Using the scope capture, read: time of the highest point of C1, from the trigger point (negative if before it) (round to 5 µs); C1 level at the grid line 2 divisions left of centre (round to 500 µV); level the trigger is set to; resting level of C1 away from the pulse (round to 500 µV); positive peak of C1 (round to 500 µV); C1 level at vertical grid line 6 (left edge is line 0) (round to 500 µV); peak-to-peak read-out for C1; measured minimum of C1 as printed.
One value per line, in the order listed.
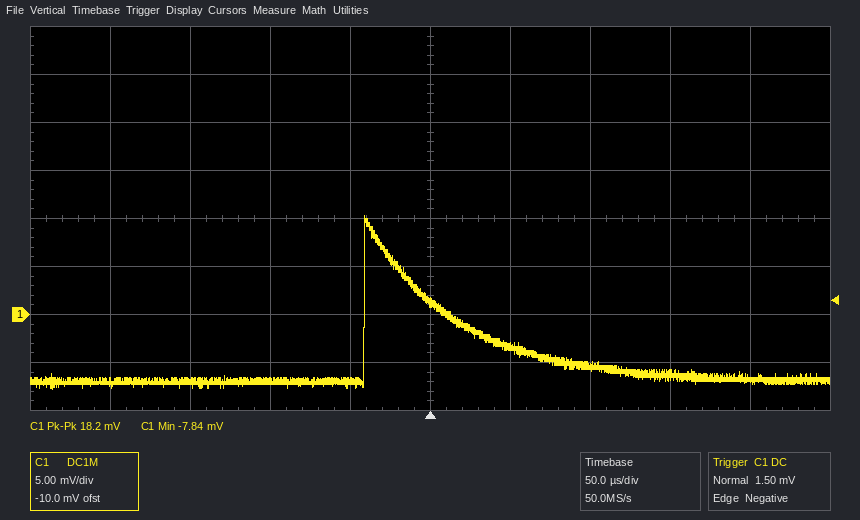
-40 µs
-7.0 mV
1.50 mV
-7.0 mV
10.5 mV
-3.5 mV
18.2 mV
-7.84 mV
